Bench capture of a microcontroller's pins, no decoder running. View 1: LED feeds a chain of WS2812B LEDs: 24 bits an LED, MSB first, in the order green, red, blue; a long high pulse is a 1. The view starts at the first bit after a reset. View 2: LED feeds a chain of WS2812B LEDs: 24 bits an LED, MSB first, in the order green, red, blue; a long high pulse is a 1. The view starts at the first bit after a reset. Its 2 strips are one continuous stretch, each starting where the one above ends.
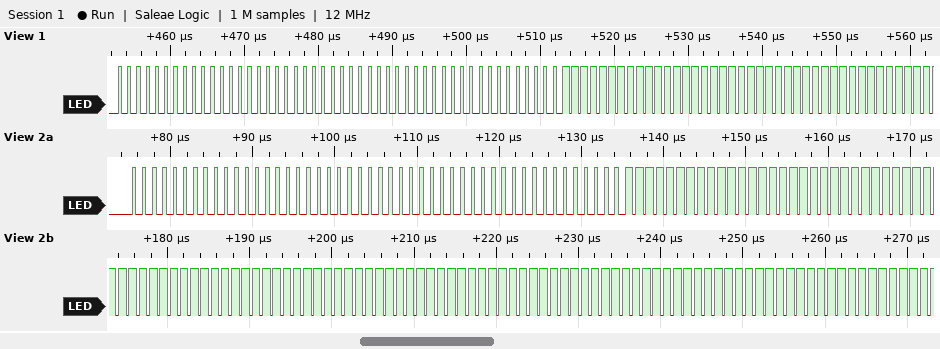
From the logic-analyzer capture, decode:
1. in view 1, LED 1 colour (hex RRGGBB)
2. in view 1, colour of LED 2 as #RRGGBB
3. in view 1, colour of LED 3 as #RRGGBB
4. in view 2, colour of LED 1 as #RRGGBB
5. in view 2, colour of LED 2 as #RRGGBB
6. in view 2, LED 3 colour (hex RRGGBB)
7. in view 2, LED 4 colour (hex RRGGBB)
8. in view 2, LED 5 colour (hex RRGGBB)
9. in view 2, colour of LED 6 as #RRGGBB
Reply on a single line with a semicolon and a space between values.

#000000; #000000; #FFFFFF; #000000; #000000; #FFFFFF; #FFFFFF; #FFFFFF; #FFFFFF
